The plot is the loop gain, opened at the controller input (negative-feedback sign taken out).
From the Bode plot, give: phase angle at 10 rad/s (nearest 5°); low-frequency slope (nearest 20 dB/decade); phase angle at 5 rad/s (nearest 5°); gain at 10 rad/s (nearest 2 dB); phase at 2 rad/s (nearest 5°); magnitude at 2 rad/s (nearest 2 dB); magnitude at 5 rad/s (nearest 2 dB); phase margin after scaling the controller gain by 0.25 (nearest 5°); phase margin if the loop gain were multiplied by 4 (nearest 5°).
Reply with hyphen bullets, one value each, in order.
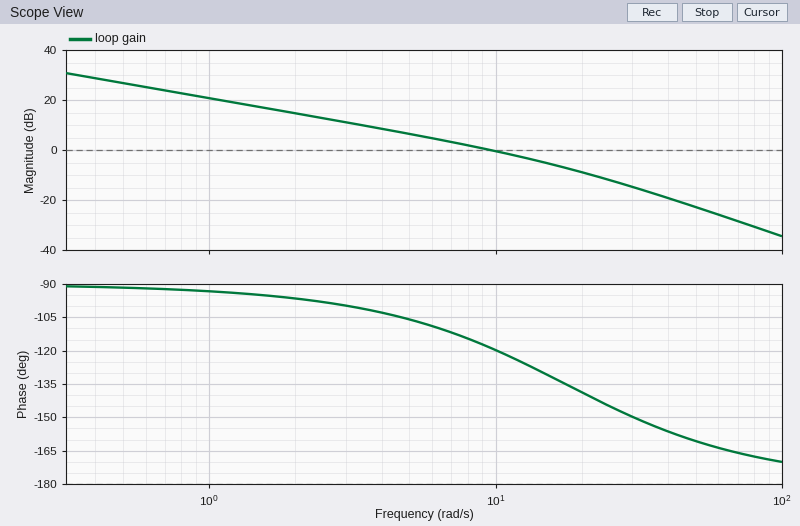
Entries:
- -120°
- -20 dB/decade
- -105°
- 0 dB
- -95°
- 14 dB
- 6 dB
- 80°
- 35°
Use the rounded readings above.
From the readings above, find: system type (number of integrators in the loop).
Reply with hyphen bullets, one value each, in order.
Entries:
- 1
